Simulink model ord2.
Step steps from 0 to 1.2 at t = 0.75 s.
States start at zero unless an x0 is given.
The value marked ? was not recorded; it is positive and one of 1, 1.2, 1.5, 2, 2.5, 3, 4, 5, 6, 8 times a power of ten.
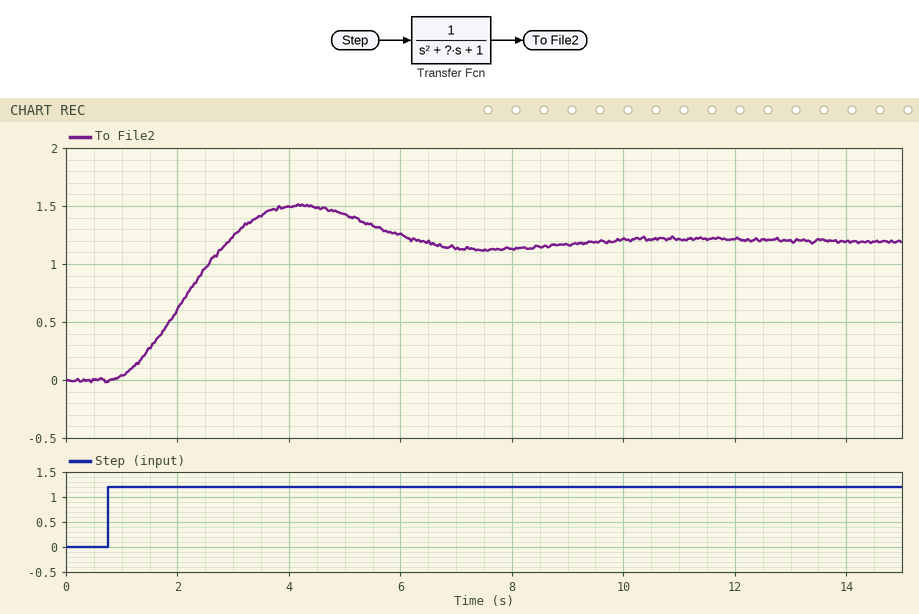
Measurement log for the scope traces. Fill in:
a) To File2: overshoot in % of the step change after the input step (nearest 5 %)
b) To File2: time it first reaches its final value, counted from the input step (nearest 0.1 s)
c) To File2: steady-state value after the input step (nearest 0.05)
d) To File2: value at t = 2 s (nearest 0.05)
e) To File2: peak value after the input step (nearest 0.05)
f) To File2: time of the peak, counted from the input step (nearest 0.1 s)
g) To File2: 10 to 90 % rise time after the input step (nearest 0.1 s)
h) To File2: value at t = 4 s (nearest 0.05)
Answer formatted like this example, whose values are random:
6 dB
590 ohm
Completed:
25 %
2.2 s
1.20
0.60
1.50
3.4 s
1.5 s
1.50
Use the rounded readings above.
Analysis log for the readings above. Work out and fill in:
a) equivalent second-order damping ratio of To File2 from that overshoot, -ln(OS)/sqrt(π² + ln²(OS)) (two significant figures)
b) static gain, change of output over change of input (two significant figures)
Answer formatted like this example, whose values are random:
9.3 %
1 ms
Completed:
0.40
1.0
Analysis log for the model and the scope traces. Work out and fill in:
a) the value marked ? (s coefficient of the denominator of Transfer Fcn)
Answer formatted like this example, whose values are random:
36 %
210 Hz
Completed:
0.8
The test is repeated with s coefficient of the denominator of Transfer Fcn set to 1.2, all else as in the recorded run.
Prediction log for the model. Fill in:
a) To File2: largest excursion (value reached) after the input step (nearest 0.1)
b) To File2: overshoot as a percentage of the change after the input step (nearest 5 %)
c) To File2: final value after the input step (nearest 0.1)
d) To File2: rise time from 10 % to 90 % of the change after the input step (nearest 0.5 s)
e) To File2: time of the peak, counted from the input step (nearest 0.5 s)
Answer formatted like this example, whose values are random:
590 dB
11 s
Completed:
1.3
10 %
1.2
2.0 s
4.0 s
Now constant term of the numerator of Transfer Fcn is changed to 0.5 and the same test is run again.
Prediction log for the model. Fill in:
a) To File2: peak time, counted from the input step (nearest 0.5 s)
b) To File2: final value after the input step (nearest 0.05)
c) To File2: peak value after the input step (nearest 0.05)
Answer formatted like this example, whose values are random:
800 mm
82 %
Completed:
3.5 s
0.60
0.75
